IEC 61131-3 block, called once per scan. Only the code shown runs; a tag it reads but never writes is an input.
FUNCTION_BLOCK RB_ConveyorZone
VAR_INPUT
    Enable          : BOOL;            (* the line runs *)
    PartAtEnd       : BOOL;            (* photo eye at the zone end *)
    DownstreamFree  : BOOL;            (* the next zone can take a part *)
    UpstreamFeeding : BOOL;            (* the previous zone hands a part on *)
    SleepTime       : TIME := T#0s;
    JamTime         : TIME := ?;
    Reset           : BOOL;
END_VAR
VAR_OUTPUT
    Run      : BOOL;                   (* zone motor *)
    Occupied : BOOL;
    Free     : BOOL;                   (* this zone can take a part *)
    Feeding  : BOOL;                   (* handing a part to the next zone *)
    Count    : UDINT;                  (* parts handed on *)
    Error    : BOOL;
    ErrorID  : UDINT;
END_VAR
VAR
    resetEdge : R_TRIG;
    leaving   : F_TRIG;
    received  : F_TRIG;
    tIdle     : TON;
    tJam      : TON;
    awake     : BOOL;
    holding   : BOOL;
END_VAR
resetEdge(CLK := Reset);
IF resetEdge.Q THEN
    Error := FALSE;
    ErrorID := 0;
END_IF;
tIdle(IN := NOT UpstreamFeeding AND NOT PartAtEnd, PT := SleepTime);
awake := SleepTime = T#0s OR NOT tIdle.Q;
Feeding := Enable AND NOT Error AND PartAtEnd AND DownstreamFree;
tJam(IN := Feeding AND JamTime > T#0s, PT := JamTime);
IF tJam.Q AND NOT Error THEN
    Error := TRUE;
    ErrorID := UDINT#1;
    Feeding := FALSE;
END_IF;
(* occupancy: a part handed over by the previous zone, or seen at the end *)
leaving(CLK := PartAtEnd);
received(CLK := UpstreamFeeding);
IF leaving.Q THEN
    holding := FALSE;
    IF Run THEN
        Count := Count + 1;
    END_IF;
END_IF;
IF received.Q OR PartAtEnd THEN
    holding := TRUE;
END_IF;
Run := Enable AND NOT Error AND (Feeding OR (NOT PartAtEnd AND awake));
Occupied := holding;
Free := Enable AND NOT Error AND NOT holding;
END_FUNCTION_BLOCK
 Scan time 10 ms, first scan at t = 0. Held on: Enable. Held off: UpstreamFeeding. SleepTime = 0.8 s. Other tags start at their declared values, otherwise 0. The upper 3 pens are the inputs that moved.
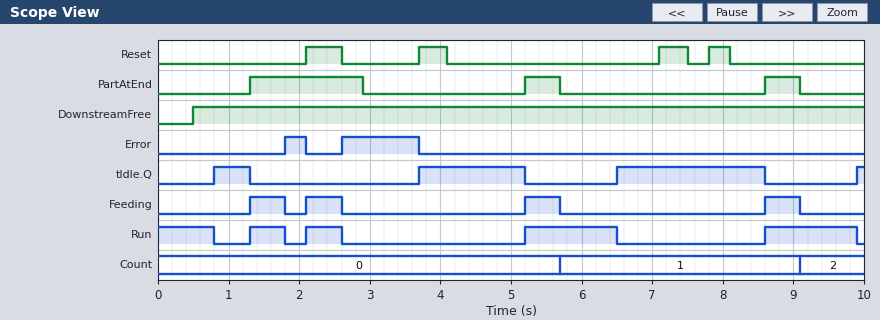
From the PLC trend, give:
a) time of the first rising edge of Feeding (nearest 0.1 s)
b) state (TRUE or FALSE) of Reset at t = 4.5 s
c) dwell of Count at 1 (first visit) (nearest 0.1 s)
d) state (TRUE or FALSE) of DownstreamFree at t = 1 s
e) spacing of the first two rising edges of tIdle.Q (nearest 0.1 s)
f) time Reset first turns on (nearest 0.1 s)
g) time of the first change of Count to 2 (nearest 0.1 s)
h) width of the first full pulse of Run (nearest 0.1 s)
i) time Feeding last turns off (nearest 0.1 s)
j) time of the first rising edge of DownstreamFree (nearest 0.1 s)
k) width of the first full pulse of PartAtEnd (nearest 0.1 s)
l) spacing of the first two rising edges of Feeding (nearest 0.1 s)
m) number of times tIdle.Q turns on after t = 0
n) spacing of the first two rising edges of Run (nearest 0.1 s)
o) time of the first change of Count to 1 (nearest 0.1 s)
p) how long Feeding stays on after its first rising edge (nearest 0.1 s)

1.3 s
FALSE
3.4 s
TRUE
2.9 s
2.1 s
9.1 s
0.5 s
9.1 s
0.5 s
1.6 s
0.8 s
4
0.8 s
5.7 s
0.5 s
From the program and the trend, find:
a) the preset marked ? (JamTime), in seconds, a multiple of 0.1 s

0.5 s
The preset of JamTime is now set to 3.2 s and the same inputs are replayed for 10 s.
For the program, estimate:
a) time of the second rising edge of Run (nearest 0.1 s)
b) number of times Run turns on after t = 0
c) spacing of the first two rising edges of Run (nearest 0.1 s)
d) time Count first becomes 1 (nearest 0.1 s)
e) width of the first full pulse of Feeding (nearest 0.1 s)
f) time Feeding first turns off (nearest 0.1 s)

5.2 s
3
3.9 s
2.9 s
1.6 s
2.9 s
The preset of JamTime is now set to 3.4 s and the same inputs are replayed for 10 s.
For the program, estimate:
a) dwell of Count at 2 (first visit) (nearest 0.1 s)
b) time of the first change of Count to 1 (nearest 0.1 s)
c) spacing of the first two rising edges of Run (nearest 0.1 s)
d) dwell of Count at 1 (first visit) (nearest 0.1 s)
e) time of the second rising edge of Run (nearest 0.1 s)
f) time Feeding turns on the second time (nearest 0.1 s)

3.4 s
2.9 s
3.9 s
2.8 s
5.2 s
5.2 s
